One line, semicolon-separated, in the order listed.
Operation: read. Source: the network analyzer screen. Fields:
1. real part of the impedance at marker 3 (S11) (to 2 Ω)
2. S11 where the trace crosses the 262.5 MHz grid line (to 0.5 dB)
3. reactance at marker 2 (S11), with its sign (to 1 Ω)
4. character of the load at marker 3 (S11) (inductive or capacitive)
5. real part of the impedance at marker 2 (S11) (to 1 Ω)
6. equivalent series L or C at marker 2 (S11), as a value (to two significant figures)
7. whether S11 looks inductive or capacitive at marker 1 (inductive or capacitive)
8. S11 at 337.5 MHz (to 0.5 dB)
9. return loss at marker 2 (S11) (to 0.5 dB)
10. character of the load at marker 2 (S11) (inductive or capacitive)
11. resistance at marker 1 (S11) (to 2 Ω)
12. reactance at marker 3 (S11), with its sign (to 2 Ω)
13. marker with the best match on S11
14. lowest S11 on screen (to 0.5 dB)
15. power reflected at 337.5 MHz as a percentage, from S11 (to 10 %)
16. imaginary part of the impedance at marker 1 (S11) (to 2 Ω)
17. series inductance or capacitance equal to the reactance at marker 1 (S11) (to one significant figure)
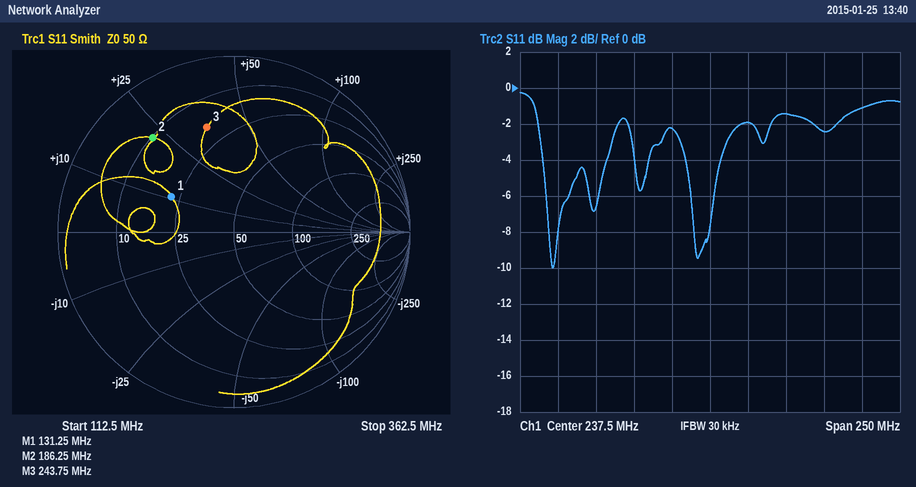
18 Ω; -2.0 dB; +22 Ω; inductive; 10 Ω; 19 nH; inductive; -1.0 dB; 3.0 dB; inductive; 22 Ω; +36 Ω; marker 1; -10.0 dB; 80 %; +10 Ω; 10 nH
